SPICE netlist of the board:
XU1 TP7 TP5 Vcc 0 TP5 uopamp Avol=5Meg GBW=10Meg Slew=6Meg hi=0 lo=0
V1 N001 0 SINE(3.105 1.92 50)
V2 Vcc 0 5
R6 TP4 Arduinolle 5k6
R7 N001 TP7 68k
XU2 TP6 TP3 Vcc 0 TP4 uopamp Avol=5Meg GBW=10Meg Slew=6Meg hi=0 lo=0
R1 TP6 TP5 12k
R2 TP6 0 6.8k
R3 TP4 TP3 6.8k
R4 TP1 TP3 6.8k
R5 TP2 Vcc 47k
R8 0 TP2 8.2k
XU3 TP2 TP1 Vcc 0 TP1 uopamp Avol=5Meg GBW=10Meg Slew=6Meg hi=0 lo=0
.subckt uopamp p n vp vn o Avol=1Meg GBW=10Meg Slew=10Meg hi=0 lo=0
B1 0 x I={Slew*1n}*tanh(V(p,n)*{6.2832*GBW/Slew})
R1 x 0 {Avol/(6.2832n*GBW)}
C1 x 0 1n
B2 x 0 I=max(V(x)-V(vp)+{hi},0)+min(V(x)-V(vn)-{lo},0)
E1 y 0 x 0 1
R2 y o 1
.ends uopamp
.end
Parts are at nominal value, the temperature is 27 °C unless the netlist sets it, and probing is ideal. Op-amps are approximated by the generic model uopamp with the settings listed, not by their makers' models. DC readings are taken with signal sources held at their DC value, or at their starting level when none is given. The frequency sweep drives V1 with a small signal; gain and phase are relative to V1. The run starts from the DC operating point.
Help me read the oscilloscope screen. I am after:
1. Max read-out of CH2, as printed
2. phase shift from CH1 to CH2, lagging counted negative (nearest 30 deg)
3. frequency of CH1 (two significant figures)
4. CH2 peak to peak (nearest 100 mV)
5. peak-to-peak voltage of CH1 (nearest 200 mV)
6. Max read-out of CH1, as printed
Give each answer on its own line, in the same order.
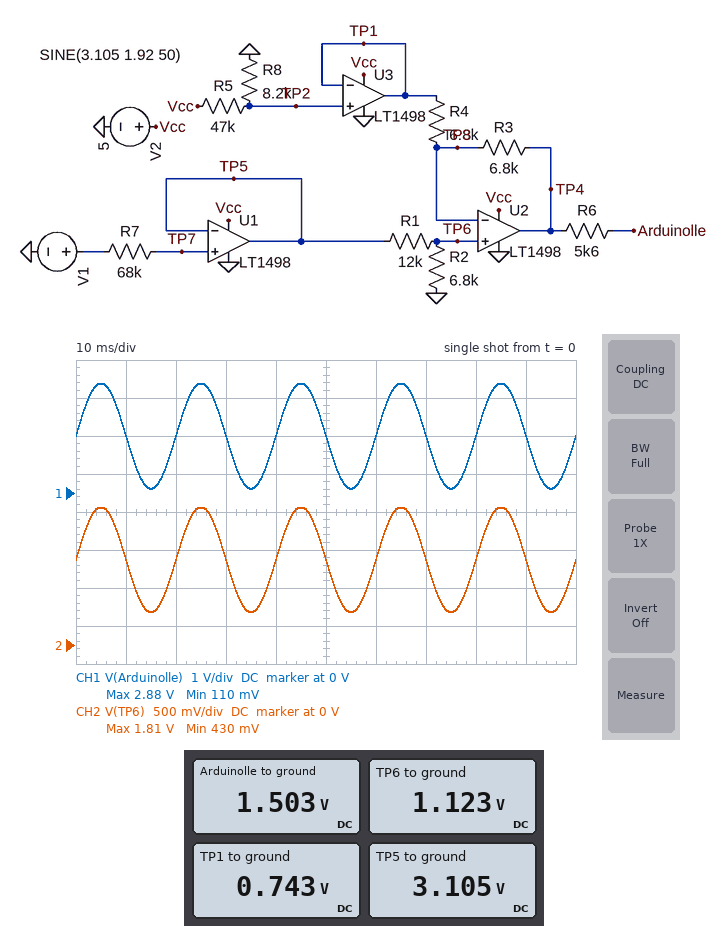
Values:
1.81 V
0 deg
50 Hz
1.4 V
2.8 V
2.88 V
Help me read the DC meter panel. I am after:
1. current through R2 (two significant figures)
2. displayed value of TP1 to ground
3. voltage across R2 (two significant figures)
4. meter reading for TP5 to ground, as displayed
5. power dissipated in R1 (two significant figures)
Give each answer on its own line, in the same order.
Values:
170 µA
0.743 V
1.1 V
3.105 V
330 µW
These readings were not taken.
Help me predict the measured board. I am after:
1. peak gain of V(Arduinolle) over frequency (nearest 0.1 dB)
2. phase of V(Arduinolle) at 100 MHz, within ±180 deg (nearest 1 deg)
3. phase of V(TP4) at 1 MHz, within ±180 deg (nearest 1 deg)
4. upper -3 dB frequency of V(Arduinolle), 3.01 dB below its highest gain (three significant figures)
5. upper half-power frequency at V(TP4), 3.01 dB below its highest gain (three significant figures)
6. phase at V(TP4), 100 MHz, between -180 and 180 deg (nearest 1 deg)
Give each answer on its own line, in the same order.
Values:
-2.8 dB
-171 deg
-17 deg
4.19 MHz
4.19 MHz
-171 deg
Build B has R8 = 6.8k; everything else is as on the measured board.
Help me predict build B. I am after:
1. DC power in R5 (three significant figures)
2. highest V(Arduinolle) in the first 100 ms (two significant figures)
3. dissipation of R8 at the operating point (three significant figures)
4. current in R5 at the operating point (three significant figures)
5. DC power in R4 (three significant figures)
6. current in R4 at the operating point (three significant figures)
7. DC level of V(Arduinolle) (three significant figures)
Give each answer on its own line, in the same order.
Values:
406 µW
3.0 V
58.7 µW
92.9 µA
35.5 µW
72.2 µA
1.61 V
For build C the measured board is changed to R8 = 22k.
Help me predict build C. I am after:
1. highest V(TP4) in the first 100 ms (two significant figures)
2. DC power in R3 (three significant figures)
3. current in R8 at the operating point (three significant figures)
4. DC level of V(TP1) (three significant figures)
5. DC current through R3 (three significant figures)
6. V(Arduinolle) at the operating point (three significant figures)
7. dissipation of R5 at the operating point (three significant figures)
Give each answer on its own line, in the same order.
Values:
2.0 V
32.6 µW
72.5 µA
1.59 V
69.3 µA
652 mV
247 µW
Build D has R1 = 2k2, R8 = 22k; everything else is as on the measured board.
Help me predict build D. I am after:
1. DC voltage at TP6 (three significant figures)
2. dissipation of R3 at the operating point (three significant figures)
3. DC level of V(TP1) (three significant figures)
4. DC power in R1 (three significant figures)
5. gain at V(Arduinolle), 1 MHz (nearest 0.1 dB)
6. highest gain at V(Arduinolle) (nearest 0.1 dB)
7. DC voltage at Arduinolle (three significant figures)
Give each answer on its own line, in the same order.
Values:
2.35 V
83.1 µW
1.59 V
262 µW
3.4 dB
3.6 dB
3.10 V
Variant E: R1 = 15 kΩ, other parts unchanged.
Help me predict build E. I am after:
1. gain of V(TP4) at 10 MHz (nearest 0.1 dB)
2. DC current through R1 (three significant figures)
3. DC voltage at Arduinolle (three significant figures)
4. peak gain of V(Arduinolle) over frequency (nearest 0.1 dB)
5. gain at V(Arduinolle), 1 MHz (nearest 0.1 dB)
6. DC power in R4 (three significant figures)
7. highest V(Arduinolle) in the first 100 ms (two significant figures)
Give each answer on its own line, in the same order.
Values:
-14.1 dB
142 µA
1.19 V
-4.1 dB
-4.3 dB
7.50 µW
2.4 V
